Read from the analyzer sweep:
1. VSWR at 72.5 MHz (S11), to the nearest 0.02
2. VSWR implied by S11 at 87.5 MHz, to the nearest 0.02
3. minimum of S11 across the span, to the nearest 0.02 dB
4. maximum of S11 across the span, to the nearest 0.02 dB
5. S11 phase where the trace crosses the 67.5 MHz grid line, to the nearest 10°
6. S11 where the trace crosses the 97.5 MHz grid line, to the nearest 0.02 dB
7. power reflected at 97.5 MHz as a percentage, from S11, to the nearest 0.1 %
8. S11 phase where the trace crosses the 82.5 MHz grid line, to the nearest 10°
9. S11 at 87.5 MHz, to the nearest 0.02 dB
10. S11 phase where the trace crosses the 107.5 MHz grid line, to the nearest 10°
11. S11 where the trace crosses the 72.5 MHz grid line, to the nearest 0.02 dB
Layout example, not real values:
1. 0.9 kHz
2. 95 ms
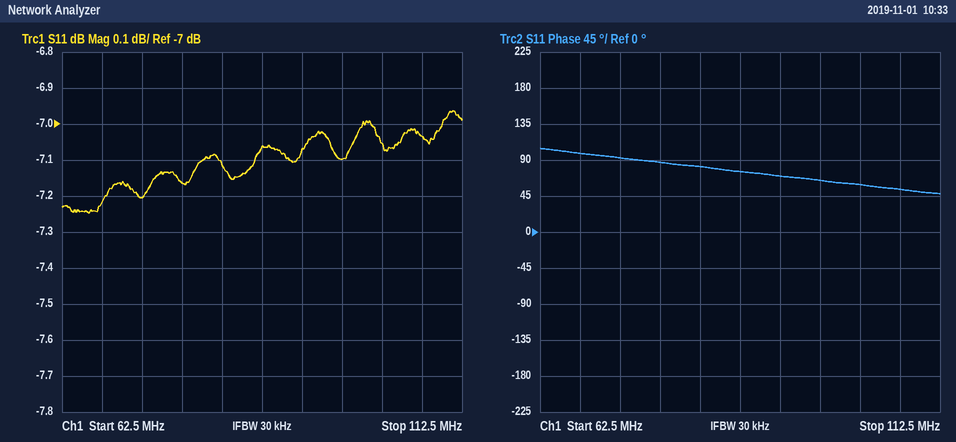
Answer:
1. 2.54
2. 2.60
3. -7.24 dB
4. -6.96 dB
5. 100°
6. -7.10 dB
7. 19.5 %
8. 80°
9. -7.06 dB
10. 50°
11. -7.20 dB
